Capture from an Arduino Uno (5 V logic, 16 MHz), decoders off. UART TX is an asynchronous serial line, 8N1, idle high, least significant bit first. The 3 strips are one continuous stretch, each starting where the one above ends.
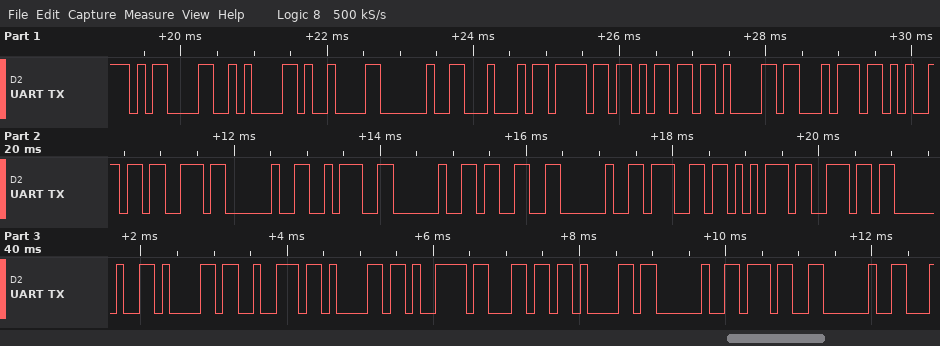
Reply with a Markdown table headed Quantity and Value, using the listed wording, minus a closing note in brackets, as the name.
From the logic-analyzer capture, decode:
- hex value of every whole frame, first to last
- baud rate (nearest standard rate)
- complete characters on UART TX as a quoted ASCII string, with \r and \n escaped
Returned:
| Quantity | Value |
|---|---|
| hex value of every whole frame, first to last | 0x0D 0x0A 0x09 0x20 0x44 0x6F 0x6D 0x61 0x74 0x65 0x73 0x20 0x3A 0x20 0x33 0x20 0x67 0x75 0x6E 0x20 0x61 0x72 0x61 0x79 0x6C 0x61 0x20 0x37 0x20 |
| baud rate | 9600 baud |
| complete characters on UART TX as a quoted ASCII string, with \r and \n escaped | "\r\n\t Domates : 3 gun arayla 7 " |
